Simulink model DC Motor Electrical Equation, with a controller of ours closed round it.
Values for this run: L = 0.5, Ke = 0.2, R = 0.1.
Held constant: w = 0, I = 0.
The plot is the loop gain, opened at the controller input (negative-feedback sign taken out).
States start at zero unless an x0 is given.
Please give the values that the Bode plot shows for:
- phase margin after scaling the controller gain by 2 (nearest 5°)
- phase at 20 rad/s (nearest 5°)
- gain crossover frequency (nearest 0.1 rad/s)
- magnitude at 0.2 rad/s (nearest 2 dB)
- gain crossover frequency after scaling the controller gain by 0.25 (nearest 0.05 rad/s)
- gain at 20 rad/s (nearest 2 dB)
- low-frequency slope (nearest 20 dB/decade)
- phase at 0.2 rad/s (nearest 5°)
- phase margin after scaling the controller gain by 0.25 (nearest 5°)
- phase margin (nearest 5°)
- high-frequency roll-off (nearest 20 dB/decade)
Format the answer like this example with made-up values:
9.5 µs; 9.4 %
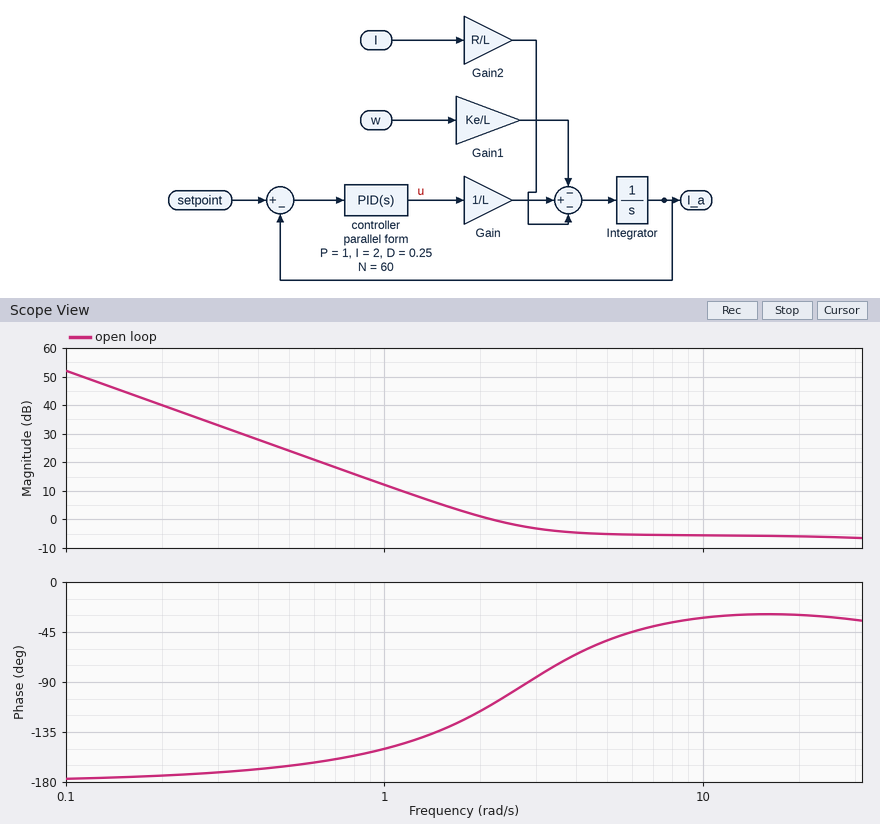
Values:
150°; -30°; 2.2 rad/s; 40 dB; 1.00 rad/s; -6 dB; -40 dB/decade; -175°; 30°; 70°; 0 dB/decade
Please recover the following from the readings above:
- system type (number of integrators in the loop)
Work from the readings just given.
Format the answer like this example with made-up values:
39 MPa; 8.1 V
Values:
2
